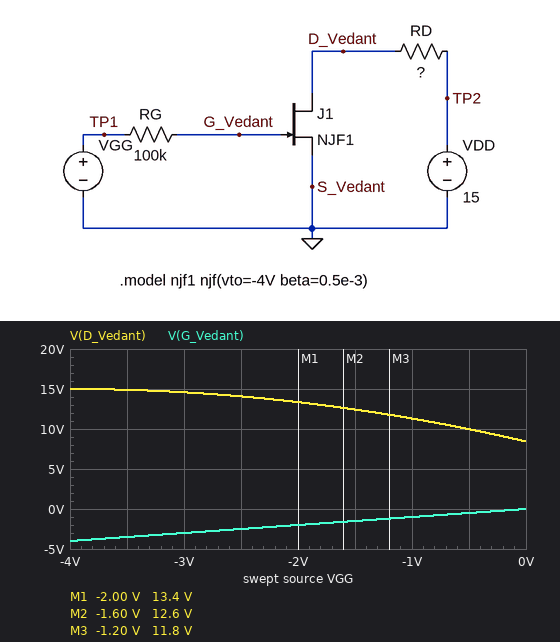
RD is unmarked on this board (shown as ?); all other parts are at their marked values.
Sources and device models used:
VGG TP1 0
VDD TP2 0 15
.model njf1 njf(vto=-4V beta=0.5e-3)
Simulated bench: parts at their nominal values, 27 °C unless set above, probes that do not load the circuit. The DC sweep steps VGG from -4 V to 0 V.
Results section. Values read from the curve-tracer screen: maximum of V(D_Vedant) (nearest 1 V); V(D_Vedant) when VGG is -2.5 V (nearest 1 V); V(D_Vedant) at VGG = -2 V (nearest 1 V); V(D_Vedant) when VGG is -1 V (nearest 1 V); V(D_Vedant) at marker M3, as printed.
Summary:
15 V
14 V
13 V
11 V
11.8 V
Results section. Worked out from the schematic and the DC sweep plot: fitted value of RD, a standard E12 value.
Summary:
820 Ω
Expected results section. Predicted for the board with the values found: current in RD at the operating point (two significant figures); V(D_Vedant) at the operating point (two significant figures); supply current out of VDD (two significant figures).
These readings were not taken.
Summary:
8.0 mA
8.4 V
8.0 mA
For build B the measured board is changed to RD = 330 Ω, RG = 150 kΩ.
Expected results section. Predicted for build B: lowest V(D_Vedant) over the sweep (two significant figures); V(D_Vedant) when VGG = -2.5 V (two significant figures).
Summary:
12 V
15 V
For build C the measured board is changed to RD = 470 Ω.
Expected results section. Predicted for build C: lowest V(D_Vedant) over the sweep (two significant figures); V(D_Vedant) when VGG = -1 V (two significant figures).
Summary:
11 V
13 V
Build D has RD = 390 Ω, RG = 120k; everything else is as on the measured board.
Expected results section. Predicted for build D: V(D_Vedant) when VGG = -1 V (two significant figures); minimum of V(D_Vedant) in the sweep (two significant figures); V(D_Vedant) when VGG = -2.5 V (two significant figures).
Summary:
13 V
12 V
15 V
